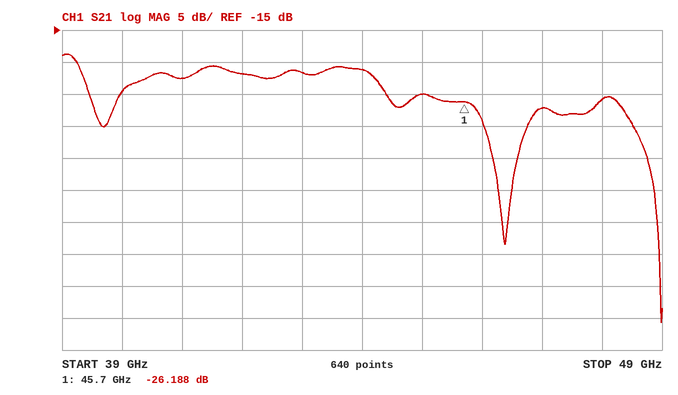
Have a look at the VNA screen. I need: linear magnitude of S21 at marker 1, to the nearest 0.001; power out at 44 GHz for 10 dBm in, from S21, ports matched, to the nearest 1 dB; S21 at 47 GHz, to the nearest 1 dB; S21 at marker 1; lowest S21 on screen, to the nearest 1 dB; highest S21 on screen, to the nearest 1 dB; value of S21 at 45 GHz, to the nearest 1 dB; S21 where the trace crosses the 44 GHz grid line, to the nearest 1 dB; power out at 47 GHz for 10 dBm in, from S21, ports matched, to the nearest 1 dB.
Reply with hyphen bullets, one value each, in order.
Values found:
- 0.049
- -11 dBm
- -27 dB
- -26.188 dB
- -61 dB
- -19 dB
- -25 dB
- -21 dB
- -17 dBm
